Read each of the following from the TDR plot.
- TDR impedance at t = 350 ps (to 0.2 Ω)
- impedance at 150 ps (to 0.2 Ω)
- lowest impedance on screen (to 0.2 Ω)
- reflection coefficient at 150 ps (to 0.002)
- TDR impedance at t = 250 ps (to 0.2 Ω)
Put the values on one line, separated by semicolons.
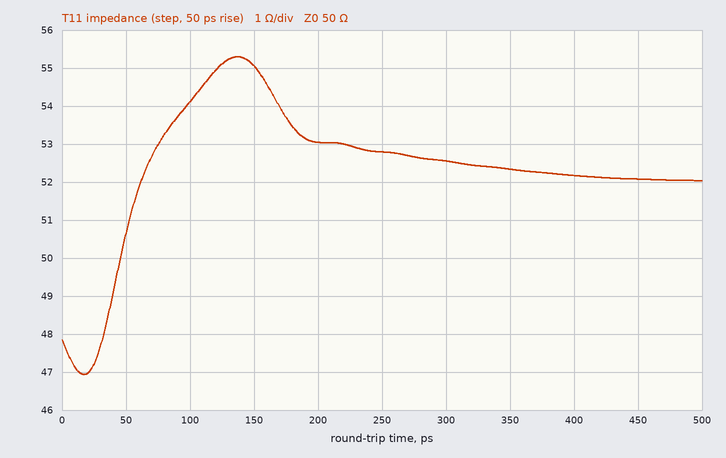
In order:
52.4 Ω; 55.0 Ω; 47.0 Ω; +0.048; 52.8 Ω
